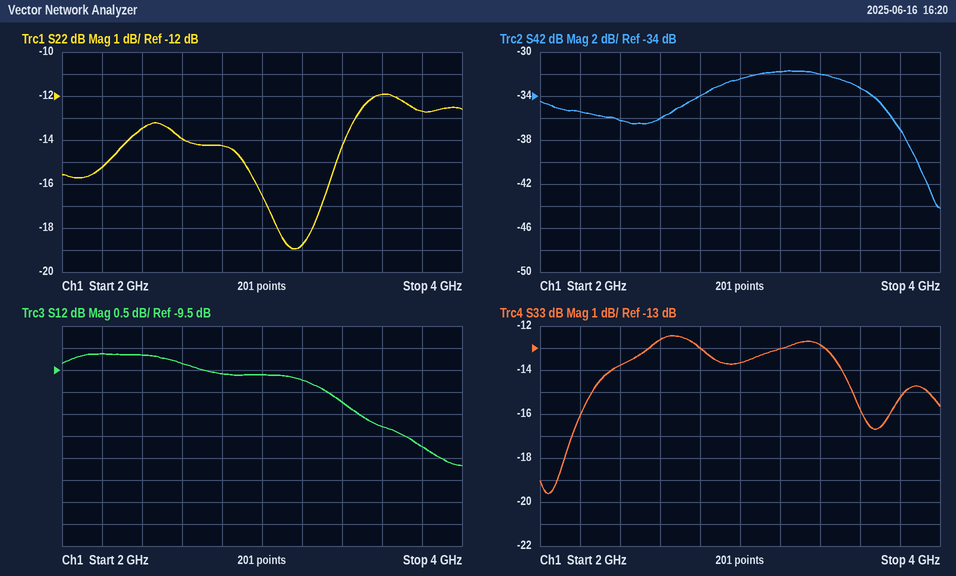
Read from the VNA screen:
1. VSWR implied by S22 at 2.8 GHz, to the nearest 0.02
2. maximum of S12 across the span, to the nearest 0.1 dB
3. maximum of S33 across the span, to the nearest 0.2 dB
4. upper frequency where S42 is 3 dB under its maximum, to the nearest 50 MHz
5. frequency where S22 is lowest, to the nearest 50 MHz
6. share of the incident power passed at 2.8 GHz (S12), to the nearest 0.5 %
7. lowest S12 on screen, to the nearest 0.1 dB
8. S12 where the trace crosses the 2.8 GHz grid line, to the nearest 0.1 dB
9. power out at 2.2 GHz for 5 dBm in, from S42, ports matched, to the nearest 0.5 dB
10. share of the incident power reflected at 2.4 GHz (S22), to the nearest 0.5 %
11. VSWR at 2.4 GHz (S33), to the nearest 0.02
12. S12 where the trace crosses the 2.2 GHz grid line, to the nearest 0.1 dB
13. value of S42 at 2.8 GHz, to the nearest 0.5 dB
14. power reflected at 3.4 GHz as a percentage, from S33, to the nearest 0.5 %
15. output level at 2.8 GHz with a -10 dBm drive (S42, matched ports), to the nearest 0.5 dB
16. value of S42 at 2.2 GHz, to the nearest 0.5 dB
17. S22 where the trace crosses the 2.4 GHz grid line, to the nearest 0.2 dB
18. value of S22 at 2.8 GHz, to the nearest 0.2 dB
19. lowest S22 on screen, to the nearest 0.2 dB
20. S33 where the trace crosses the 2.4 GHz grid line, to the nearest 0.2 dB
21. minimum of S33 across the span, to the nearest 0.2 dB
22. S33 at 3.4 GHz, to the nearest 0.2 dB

1.48
-9.1 dB
-12.4 dB
3.70 GHz
3.15 GHz
11.0 %
-11.7 dB
-9.6 dB
-30.5 dBm
4.5 %
1.52
-9.1 dB
-34.0 dB
5.0 %
-44.0 dBm
-35.5 dB
-13.4 dB
-14.2 dB
-19.0 dB
-13.8 dB
-19.6 dB
-12.8 dB
